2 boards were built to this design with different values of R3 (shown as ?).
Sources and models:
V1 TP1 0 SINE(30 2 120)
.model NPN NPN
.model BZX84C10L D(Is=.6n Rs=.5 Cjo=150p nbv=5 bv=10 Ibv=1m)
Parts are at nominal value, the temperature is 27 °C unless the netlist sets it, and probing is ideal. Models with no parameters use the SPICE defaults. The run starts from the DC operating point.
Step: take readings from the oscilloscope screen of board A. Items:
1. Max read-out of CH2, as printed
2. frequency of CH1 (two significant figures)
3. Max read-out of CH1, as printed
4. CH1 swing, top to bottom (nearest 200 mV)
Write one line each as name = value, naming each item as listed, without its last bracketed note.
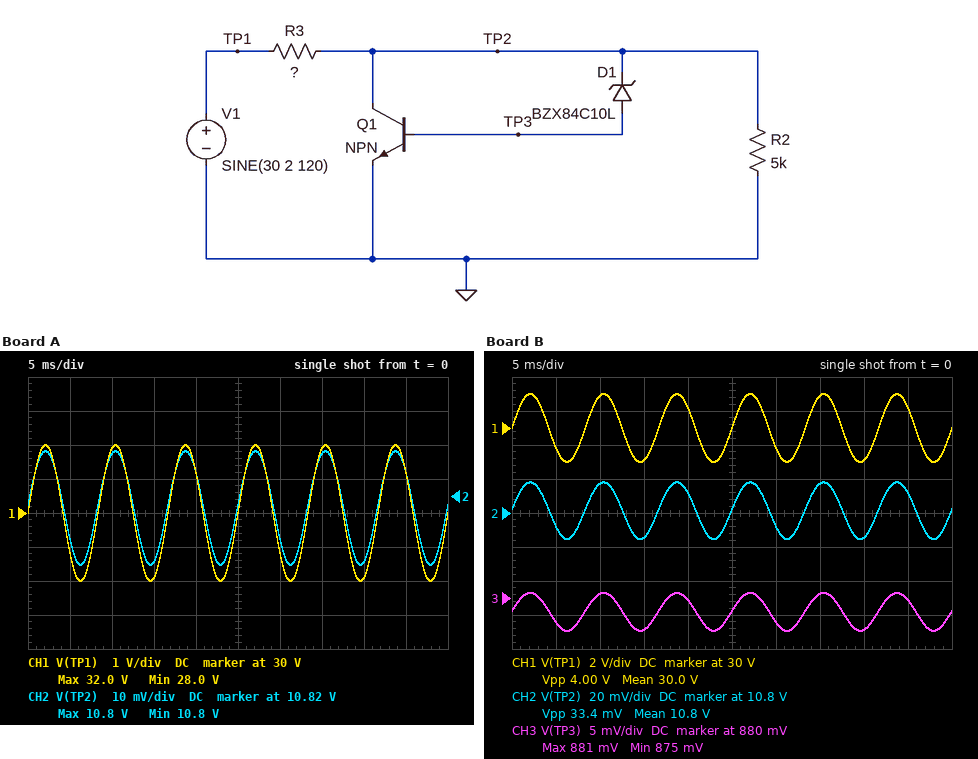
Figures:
Max read-out of CH2, as printed = 10.8 V
frequency of CH1 = 120 Hz
Max read-out of CH1, as printed = 32.0 V
CH1 swing, top to bottom = 4.0 V
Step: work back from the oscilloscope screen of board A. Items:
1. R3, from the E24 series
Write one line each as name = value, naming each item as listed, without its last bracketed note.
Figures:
R3, from the E24 series = 300 Ω
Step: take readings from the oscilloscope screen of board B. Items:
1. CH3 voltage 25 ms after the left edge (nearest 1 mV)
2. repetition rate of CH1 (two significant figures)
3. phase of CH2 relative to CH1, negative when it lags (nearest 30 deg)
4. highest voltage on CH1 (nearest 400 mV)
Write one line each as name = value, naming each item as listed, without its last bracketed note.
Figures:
CH3 voltage 25 ms after the left edge = 878 mV
repetition rate of CH1 = 120 Hz
phase of CH2 relative to CH1, negative when it lags = 0 deg
highest voltage on CH1 = 32.0 V
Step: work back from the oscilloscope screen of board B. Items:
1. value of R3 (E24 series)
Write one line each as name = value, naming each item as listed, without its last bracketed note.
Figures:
value of R3 = 330 Ω
